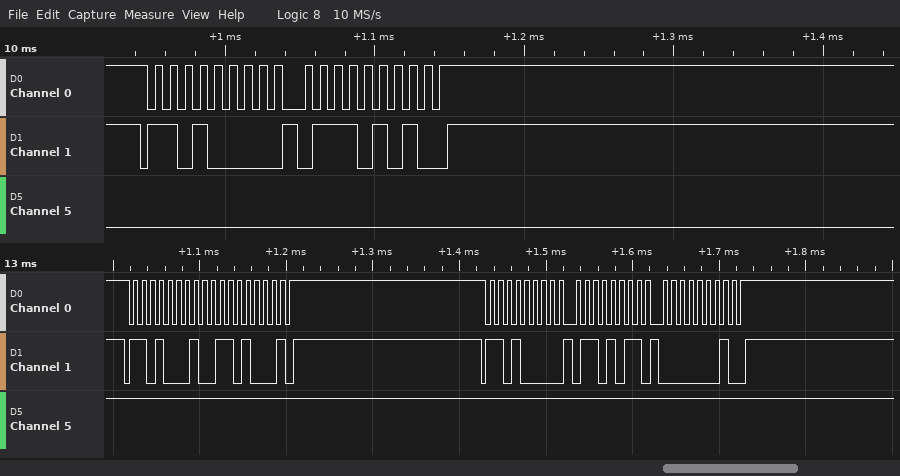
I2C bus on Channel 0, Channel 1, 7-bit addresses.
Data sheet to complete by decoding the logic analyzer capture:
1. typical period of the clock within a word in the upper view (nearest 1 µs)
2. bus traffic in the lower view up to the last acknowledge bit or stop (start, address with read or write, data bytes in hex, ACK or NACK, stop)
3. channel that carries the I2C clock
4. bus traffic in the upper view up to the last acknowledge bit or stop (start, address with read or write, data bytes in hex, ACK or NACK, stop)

10 µs
start, address 68 read ACK, 68 NACK, stop, start, address 68 write ACK, 6B ACK, 01 ACK, stop
Channel 0
start, address 68 write ACK, 75 ACK, stop
